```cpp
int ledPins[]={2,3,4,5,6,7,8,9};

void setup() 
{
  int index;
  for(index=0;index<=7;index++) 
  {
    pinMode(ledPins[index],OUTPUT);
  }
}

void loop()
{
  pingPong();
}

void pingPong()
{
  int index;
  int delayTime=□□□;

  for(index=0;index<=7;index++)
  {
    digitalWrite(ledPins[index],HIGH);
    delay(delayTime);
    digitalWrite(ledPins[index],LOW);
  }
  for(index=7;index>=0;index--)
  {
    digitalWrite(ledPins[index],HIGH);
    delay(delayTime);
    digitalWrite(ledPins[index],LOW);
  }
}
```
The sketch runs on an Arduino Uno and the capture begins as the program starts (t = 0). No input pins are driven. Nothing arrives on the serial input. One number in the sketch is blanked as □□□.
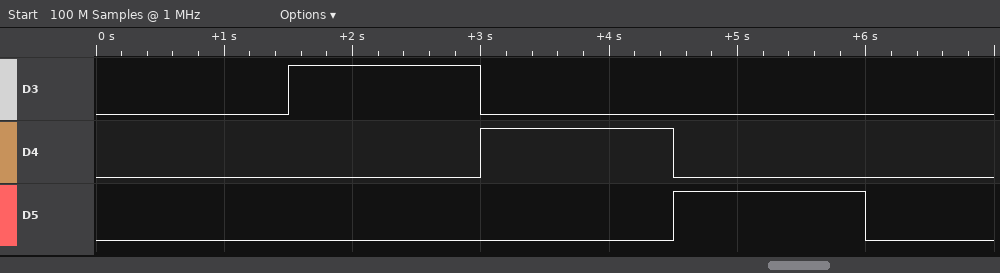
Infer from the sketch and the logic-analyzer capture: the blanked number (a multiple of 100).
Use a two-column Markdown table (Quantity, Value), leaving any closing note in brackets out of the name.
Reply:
| Quantity | Value |
|---|---|
| the blanked number | 1500 |
